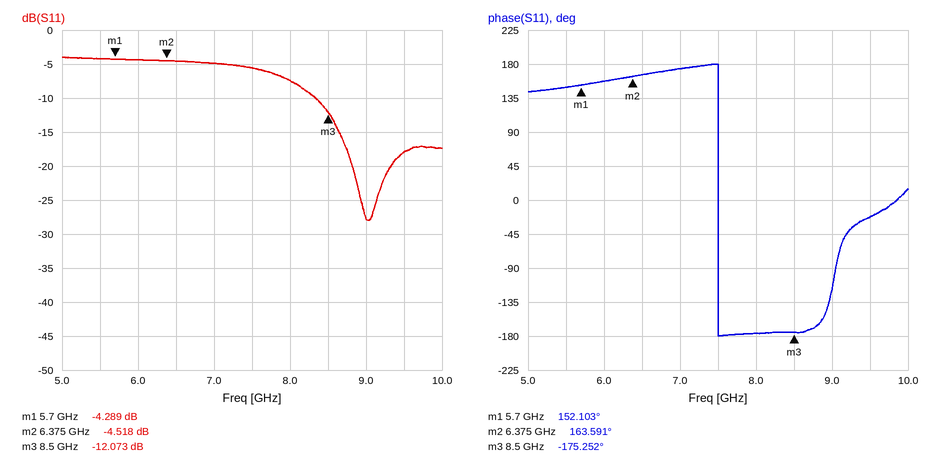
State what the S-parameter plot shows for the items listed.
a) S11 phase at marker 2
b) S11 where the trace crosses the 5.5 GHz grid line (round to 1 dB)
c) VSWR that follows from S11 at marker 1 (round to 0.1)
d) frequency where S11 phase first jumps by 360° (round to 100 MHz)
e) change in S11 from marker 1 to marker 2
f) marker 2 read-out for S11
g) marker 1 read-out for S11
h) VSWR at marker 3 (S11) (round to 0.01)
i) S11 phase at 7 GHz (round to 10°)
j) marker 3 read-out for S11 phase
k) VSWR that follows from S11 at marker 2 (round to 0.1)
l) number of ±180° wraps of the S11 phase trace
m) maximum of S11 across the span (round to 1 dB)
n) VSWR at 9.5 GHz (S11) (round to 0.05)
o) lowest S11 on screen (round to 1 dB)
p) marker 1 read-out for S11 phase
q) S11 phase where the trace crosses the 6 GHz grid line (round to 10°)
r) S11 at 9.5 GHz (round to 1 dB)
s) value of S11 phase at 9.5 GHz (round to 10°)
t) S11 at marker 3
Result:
163.591°
-4 dB
4.1
7.5 GHz
-0.229 dB
-4.518 dB
-4.289 dB
1.66
170°
-175.252°
3.9
1
-4 dB
1.30
-28 dB
152.103°
160°
-18 dB
-20°
-12.073 dB
